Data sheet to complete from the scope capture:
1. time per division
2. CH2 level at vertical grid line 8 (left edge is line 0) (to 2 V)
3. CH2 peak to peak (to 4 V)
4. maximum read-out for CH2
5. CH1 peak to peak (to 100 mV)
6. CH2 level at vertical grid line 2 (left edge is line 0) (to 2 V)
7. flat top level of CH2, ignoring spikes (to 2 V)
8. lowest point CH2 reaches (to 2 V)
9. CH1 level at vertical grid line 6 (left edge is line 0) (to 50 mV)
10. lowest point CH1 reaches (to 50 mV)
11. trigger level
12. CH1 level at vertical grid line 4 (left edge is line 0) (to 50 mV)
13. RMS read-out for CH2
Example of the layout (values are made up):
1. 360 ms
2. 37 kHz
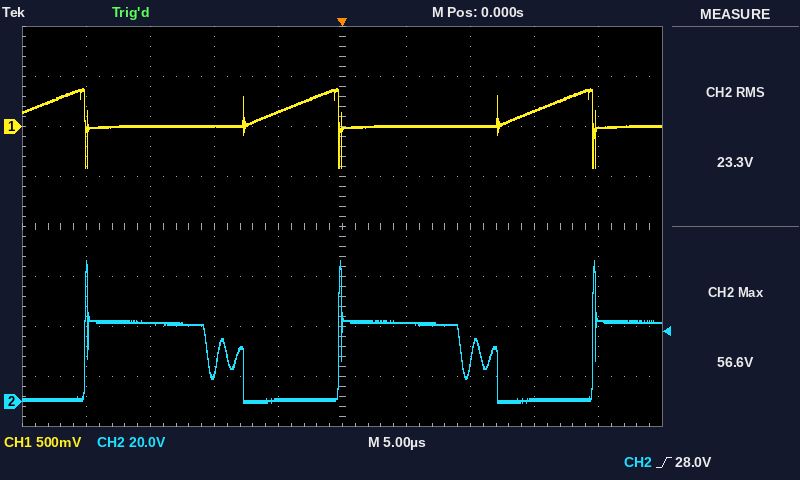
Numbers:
1. 5 µs
2. 0 V
3. 56 V
4. 56.6 V
5. 800 mV
6. 32 V
7. 32 V
8. 0 V
9. 0 mV
10. -400 mV
11. 28.0 V
12. 150 mV
13. 23.3 V
